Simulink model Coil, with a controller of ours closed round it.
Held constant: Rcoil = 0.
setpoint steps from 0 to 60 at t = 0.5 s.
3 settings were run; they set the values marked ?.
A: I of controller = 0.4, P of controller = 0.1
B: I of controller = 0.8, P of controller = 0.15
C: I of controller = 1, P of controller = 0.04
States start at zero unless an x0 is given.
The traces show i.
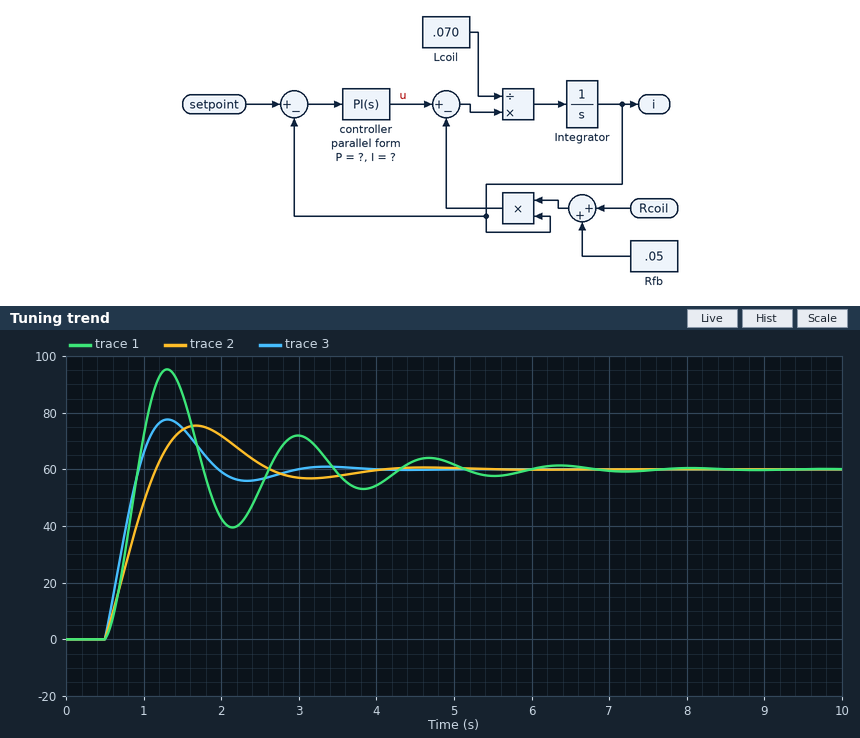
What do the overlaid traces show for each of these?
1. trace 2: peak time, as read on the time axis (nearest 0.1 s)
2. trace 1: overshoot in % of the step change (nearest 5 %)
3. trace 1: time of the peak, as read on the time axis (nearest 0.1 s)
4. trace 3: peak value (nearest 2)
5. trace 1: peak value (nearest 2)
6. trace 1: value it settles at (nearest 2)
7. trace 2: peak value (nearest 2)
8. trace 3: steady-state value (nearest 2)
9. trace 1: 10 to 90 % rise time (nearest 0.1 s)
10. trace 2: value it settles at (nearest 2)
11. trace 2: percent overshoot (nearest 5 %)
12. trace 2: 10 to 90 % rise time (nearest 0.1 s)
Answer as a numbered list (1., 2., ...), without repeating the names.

1. 1.7 s
2. 60 %
3. 1.3 s
4. 78
5. 96
6. 60
7. 76
8. 60
9. 0.3 s
10. 60
11. 25 %
12. 0.5 s
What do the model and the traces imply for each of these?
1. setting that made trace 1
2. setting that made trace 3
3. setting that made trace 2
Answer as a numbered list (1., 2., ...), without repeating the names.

1. C
2. B
3. A
